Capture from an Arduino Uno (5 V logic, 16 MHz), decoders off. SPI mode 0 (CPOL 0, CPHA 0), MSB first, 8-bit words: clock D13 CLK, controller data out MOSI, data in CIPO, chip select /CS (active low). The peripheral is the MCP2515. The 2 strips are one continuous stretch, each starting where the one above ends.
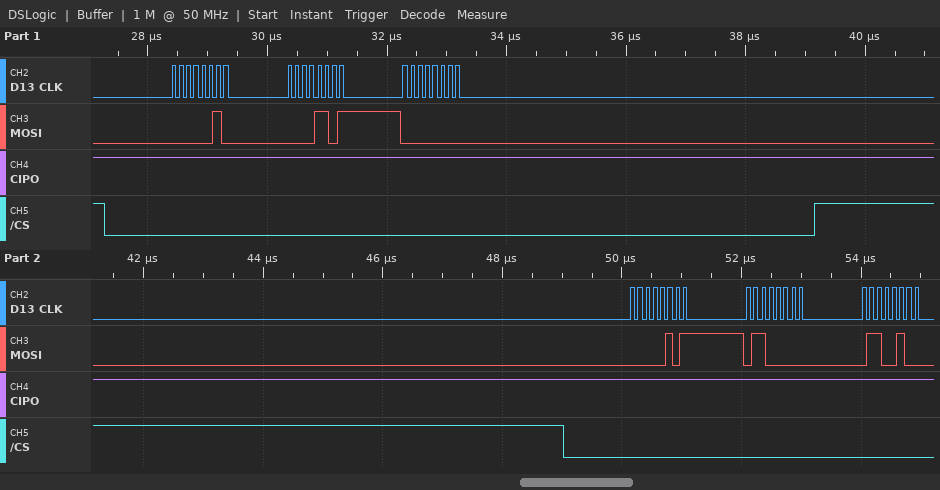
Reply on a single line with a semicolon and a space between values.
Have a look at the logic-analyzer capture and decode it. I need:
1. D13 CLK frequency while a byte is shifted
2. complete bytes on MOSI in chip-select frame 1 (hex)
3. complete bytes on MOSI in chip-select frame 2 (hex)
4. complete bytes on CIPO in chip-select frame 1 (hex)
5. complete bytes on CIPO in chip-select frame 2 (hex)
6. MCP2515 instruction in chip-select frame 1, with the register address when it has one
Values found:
8 MHz; 02 0D 00; 05 60 64; FF FF FF; FF FF FF; WRITE 0x0D
